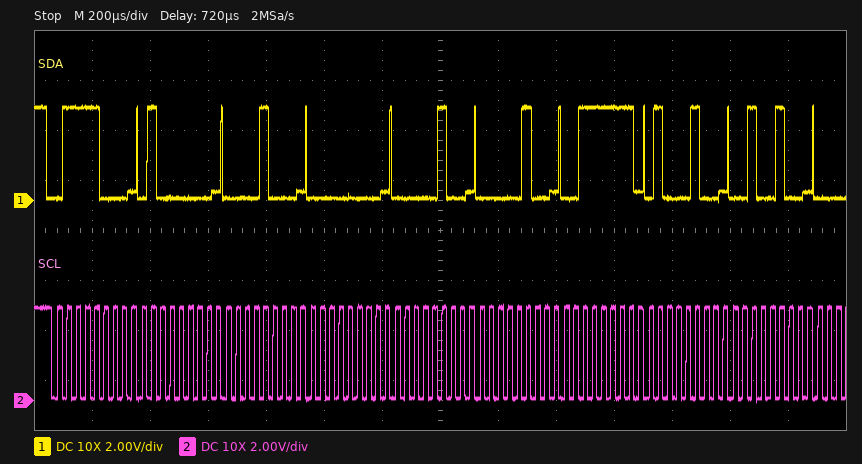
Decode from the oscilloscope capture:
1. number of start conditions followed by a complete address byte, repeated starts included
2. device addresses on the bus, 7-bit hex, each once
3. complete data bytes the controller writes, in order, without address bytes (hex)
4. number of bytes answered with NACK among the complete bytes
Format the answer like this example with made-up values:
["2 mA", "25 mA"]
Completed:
["1", "0x3C", "40 08 00 04 04 3F 44 24", "0"]
